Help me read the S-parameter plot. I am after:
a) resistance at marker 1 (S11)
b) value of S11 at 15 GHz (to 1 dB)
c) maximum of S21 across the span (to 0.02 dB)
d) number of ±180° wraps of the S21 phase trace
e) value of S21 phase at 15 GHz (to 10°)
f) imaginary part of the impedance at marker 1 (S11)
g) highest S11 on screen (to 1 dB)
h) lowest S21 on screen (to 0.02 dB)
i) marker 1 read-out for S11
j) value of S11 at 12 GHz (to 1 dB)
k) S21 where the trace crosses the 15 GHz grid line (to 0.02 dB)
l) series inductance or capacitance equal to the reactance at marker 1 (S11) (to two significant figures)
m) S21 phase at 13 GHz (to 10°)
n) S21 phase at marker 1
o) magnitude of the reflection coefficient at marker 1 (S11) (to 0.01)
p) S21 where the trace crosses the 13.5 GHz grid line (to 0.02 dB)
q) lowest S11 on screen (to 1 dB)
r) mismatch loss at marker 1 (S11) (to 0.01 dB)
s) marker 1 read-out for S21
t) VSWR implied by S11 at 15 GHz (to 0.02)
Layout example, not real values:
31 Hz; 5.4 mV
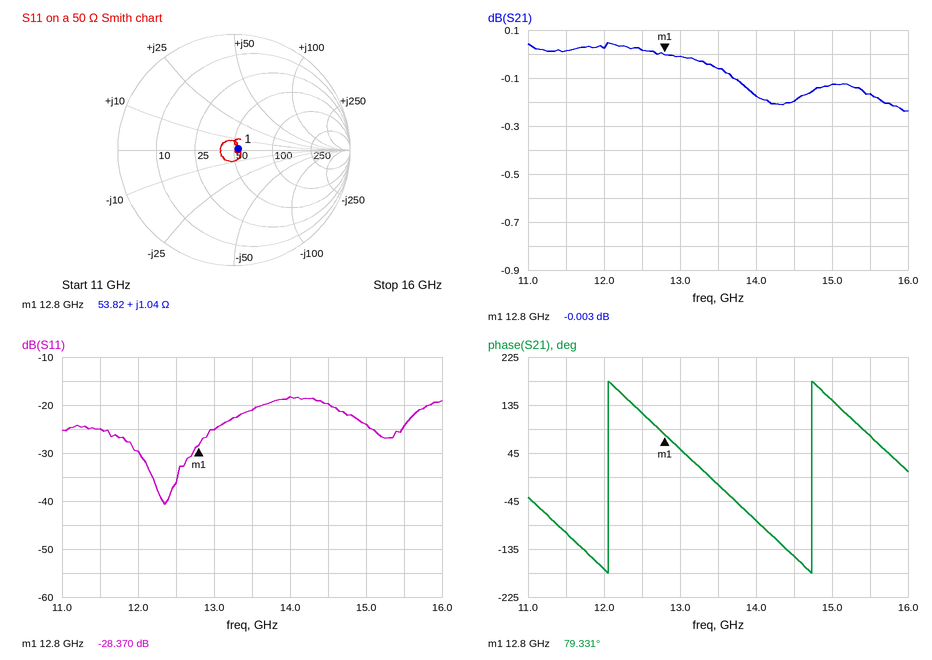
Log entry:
53.82 Ω; -24 dB; 0.04 dB; 2; 140°; +1.04 Ω; -18 dB; -0.24 dB; -28.370 dB; -30 dB; -0.12 dB; 13 pH; 50°; 79.331°; 0.04; -0.06 dB; -41 dB; 0.01 dB; -0.003 dB; 1.14
